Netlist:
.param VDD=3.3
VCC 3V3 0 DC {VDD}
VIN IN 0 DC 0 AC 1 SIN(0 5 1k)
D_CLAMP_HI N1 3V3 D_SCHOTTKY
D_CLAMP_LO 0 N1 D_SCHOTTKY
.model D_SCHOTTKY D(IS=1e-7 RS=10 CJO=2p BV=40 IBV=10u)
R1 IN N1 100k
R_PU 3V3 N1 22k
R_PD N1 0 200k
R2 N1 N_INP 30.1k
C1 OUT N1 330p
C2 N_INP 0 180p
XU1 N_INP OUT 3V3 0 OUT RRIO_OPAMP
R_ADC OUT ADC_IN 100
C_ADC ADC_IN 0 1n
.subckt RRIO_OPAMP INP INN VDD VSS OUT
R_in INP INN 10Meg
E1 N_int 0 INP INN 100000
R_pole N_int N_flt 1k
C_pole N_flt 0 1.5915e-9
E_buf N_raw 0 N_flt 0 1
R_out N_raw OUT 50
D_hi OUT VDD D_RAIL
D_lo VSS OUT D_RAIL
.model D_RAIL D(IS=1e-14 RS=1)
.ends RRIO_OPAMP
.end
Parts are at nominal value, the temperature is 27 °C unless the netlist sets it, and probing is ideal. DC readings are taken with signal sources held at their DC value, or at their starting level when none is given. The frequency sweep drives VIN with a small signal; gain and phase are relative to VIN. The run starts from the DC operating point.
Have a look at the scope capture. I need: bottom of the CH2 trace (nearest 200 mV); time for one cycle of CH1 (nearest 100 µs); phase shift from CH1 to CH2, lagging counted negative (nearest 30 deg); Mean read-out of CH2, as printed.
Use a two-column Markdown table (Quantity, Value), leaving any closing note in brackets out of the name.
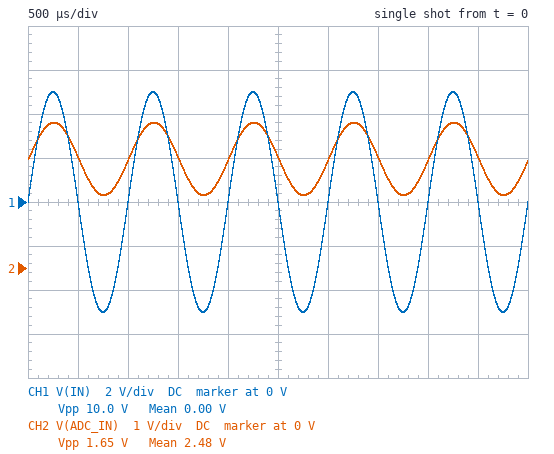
| Quantity | Value |
|---|---|
| bottom of the CH2 trace | 1.6 V |
| time for one cycle of CH1 | 1.0 ms |
| phase shift from CH1 to CH2, lagging counted negative | 0 deg |
| Mean read-out of CH2, as printed | 2.48 V |
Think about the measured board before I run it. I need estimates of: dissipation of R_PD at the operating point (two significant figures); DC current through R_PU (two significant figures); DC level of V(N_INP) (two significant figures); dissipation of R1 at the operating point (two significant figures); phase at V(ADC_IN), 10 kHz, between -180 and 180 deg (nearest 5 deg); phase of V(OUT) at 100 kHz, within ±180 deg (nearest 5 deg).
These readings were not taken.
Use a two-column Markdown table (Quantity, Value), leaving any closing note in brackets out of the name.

| Quantity | Value |
|---|---|
| dissipation of R_PD at the operating point | 31 µW |
| DC current through R_PU | 37 µA |
| DC level of V(N_INP) | 2.5 V |
| dissipation of R1 at the operating point | 62 µW |
| phase at V(ADC_IN), 10 kHz, between -180 and 180 deg | -30 deg |
| phase of V(OUT) at 100 kHz, within ±180 deg | -155 deg |
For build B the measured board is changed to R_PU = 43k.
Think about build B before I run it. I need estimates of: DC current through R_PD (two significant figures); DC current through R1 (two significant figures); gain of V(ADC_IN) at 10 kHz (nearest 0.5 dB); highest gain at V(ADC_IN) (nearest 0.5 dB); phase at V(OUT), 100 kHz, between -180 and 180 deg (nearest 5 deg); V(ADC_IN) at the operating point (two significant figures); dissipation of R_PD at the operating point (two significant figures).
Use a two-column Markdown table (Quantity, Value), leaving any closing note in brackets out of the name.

| Quantity | Value |
|---|---|
| DC current through R_PD | 10 µA |
| DC current through R1 | 20 µA |
| gain of V(ADC_IN) at 10 kHz | -12.0 dB |
| highest gain at V(ADC_IN) | -11.5 dB |
| phase at V(OUT), 100 kHz, between -180 and 180 deg | -160 deg |
| V(ADC_IN) at the operating point | 2.0 V |
| dissipation of R_PD at the operating point | 20 µW |
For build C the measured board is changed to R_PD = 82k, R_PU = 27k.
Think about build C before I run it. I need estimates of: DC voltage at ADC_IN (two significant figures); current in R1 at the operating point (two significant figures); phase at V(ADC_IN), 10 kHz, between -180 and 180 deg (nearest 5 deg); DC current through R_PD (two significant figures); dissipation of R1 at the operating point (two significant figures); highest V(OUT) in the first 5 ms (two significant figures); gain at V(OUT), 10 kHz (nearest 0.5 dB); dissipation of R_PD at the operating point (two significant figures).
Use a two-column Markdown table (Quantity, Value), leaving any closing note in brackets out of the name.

| Quantity | Value |
|---|---|
| DC voltage at ADC_IN | 2.1 V |
| current in R1 at the operating point | 21 µA |
| phase at V(ADC_IN), 10 kHz, between -180 and 180 deg | -30 deg |
| DC current through R_PD | 25 µA |
| dissipation of R1 at the operating point | 43 µW |
| highest V(OUT) in the first 5 ms | 2.9 V |
| gain at V(OUT), 10 kHz | -15.5 dB |
| dissipation of R_PD at the operating point | 52 µW |
